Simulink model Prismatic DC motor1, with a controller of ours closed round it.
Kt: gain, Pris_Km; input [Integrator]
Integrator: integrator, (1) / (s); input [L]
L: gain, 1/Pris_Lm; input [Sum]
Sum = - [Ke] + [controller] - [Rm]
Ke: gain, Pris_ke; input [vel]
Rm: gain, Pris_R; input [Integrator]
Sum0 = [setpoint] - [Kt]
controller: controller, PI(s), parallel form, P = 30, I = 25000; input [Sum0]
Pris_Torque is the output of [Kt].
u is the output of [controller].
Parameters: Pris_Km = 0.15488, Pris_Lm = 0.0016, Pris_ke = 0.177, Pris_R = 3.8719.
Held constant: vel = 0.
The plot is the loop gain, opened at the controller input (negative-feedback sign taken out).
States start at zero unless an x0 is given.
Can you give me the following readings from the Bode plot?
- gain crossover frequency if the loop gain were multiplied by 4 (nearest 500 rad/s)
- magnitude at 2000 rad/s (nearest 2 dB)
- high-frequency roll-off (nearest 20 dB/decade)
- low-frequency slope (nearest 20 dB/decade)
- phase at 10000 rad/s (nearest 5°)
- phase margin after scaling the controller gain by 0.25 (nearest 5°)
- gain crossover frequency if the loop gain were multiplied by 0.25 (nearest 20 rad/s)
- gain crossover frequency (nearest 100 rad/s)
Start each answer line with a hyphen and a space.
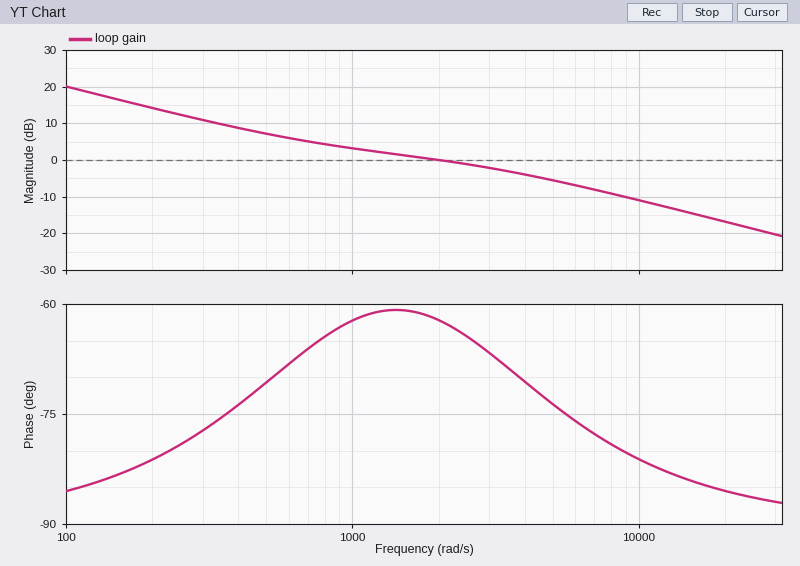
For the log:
- 11500 rad/s
- 0 dB
- -20 dB/decade
- -20 dB/decade
- -80°
- 100°
- 260 rad/s
- 2000 rad/s
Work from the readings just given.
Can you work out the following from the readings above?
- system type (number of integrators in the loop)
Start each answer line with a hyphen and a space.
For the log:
- 1
